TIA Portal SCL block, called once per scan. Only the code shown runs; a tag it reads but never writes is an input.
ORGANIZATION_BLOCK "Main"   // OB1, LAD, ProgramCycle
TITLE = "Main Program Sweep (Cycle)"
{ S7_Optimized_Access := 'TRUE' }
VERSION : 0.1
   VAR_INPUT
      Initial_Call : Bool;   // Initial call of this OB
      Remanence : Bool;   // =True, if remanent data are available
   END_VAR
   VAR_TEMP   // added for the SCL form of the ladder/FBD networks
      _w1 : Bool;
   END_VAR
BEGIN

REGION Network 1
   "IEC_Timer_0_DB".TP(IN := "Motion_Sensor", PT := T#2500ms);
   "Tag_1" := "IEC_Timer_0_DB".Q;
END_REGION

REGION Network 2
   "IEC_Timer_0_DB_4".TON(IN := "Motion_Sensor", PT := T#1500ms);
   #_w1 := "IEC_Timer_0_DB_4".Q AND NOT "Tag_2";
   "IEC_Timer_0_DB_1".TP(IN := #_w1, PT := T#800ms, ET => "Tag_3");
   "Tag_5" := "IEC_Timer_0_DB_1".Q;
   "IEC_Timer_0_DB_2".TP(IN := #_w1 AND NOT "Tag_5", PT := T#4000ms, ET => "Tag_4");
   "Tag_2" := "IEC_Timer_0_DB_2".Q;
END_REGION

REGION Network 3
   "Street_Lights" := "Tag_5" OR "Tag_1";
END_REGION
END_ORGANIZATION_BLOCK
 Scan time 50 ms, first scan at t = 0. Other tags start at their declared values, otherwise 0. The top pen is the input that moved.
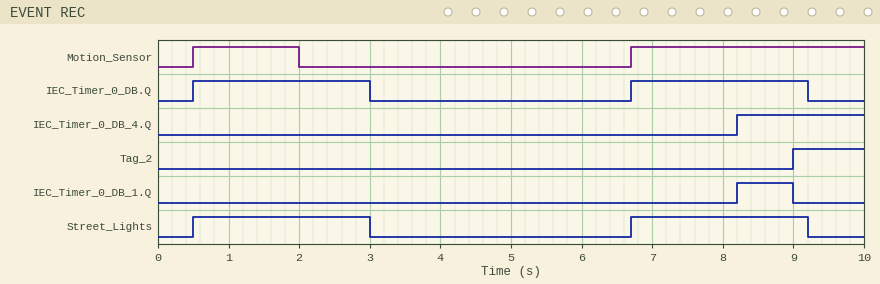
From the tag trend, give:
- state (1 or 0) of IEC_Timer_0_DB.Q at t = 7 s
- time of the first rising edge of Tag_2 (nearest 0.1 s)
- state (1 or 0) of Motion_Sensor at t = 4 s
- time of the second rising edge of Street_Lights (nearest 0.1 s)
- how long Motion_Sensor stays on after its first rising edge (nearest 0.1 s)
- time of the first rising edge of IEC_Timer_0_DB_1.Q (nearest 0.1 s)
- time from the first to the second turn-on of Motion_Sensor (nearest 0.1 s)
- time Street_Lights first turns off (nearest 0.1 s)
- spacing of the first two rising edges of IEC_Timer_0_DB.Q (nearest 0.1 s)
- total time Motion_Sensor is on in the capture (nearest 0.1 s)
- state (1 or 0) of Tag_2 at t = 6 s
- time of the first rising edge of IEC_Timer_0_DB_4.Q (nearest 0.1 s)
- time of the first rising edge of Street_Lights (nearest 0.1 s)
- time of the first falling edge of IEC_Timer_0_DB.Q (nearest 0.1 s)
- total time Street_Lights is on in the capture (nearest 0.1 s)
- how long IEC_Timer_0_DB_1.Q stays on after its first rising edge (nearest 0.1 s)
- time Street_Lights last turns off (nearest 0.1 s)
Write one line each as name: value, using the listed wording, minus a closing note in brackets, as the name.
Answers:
state (1 or 0) of IEC_Timer_0_DB.Q at t = 7 s: 1
time of the first rising edge of Tag_2: 9.0 s
state (1 or 0) of Motion_Sensor at t = 4 s: 0
time of the second rising edge of Street_Lights: 6.7 s
how long Motion_Sensor stays on after its first rising edge: 1.5 s
time of the first rising edge of IEC_Timer_0_DB_1.Q: 8.2 s
time from the first to the second turn-on of Motion_Sensor: 6.2 s
time Street_Lights first turns off: 3.0 s
spacing of the first two rising edges of IEC_Timer_0_DB.Q: 6.2 s
total time Motion_Sensor is on in the capture: 4.8 s
state (1 or 0) of Tag_2 at t = 6 s: 0
time of the first rising edge of IEC_Timer_0_DB_4.Q: 8.2 s
time of the first rising edge of Street_Lights: 0.5 s
time of the first falling edge of IEC_Timer_0_DB.Q: 3.0 s
total time Street_Lights is on in the capture: 5.0 s
how long IEC_Timer_0_DB_1.Q stays on after its first rising edge: 0.8 s
time Street_Lights last turns off: 9.2 s
